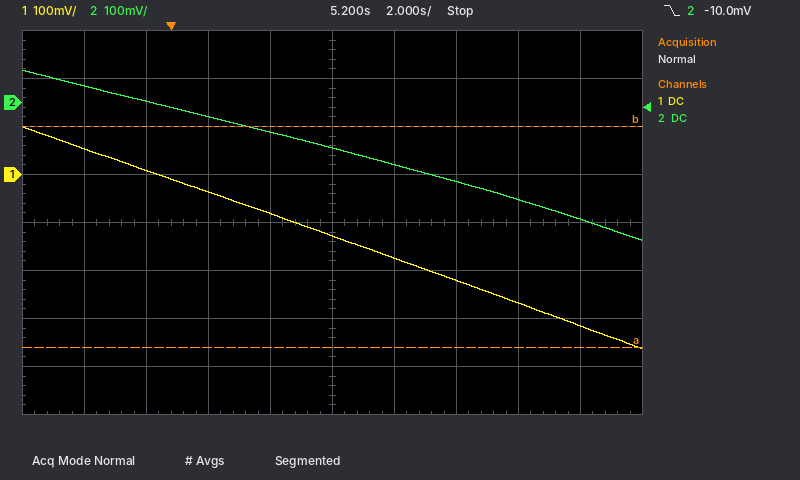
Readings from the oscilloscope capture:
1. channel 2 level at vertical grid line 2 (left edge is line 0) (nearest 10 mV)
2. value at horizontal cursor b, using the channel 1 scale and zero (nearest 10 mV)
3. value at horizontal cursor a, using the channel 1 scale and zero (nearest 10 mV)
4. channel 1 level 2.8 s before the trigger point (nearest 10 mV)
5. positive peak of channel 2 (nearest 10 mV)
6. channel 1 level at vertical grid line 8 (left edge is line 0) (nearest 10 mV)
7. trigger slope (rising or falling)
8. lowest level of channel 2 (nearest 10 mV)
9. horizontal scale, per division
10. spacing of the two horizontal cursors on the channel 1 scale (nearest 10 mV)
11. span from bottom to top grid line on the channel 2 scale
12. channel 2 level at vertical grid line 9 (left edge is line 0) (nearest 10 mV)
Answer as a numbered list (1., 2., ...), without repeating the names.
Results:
1. 0 mV
2. 100 mV
3. -360 mV
4. 50 mV
5. 70 mV
6. -270 mV
7. falling
8. -290 mV
9. 2 s
10. 460 mV
11. 800 mV
12. -240 mV
